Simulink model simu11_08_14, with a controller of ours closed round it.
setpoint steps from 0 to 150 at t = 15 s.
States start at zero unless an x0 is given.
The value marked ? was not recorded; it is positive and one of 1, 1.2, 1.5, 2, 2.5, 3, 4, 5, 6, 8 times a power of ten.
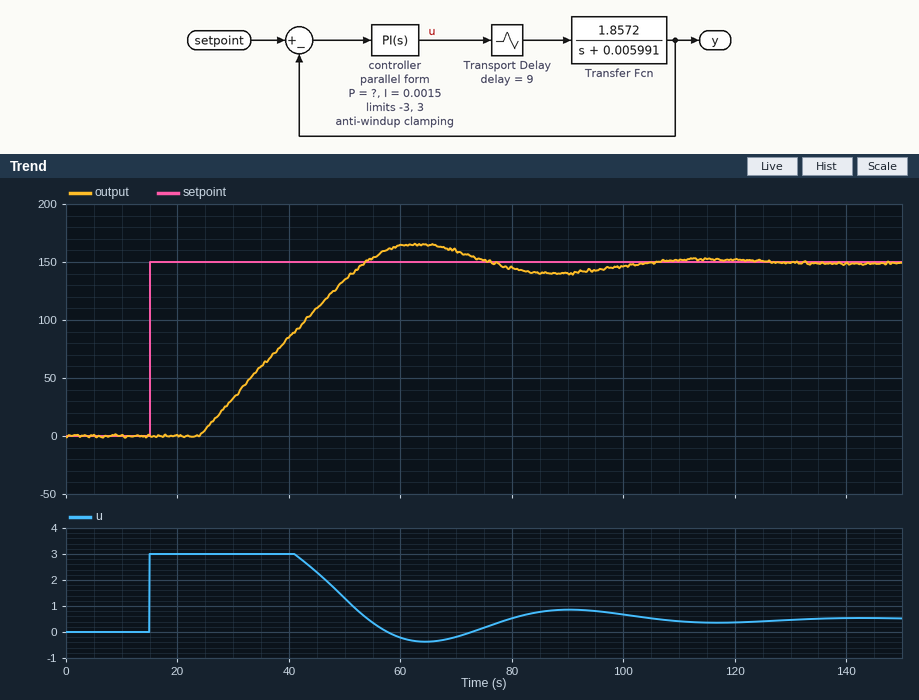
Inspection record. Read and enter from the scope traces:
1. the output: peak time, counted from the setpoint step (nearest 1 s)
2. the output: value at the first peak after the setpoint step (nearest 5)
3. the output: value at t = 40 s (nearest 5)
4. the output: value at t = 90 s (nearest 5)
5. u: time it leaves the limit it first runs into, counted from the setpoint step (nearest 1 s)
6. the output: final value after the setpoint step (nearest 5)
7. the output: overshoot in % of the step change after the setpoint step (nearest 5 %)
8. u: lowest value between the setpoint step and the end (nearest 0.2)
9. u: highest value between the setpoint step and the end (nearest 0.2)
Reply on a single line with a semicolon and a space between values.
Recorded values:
48 s; 165; 85; 140; 26 s; 150; 10 %; -0.4; 3.0
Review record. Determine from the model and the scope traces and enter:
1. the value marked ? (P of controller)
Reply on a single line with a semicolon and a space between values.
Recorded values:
0.05
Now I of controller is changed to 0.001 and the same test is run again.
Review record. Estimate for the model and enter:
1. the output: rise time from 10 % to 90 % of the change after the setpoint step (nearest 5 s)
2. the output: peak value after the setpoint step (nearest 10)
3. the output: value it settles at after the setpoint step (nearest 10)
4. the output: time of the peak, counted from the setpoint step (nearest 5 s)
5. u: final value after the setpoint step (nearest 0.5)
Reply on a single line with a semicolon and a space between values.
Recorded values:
25 s; 160; 150; 45 s; 0.5
